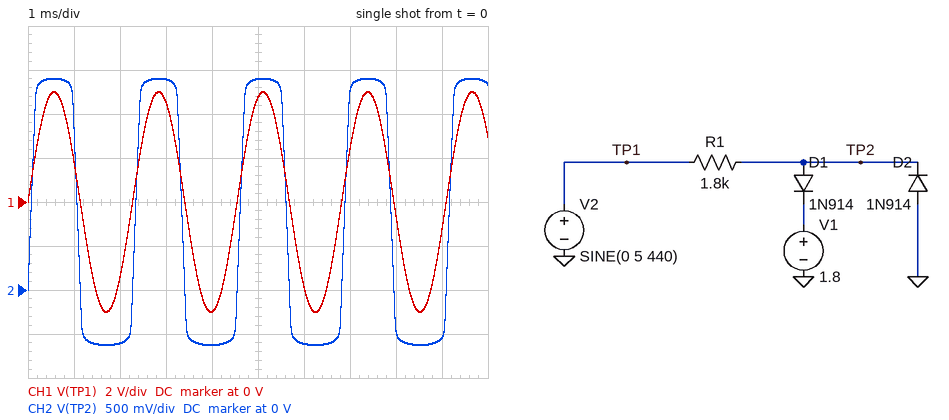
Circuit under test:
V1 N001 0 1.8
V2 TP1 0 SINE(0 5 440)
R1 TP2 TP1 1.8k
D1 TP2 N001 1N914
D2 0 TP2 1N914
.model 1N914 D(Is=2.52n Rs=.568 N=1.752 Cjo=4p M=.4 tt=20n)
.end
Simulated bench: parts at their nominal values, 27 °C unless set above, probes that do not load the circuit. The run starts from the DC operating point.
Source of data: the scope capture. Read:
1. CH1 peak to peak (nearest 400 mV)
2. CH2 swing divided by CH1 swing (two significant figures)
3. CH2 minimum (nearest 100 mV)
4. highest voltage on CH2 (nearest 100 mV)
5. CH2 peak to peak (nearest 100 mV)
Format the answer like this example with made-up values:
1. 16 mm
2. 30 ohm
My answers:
1. 10.0 V
2. 0.30
3. -600 mV
4. 2.4 V
5. 3.0 V
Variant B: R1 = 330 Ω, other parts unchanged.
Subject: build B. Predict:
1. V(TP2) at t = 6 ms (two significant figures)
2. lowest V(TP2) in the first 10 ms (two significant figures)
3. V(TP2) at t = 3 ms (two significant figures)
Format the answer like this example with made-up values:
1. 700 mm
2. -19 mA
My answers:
1. -690 mV
2. -710 mV
3. 2.5 V
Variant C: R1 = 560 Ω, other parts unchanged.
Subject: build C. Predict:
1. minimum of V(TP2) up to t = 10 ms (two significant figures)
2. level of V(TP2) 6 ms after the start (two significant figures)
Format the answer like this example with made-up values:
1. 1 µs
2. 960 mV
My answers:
1. -680 mV
2. -670 mV
